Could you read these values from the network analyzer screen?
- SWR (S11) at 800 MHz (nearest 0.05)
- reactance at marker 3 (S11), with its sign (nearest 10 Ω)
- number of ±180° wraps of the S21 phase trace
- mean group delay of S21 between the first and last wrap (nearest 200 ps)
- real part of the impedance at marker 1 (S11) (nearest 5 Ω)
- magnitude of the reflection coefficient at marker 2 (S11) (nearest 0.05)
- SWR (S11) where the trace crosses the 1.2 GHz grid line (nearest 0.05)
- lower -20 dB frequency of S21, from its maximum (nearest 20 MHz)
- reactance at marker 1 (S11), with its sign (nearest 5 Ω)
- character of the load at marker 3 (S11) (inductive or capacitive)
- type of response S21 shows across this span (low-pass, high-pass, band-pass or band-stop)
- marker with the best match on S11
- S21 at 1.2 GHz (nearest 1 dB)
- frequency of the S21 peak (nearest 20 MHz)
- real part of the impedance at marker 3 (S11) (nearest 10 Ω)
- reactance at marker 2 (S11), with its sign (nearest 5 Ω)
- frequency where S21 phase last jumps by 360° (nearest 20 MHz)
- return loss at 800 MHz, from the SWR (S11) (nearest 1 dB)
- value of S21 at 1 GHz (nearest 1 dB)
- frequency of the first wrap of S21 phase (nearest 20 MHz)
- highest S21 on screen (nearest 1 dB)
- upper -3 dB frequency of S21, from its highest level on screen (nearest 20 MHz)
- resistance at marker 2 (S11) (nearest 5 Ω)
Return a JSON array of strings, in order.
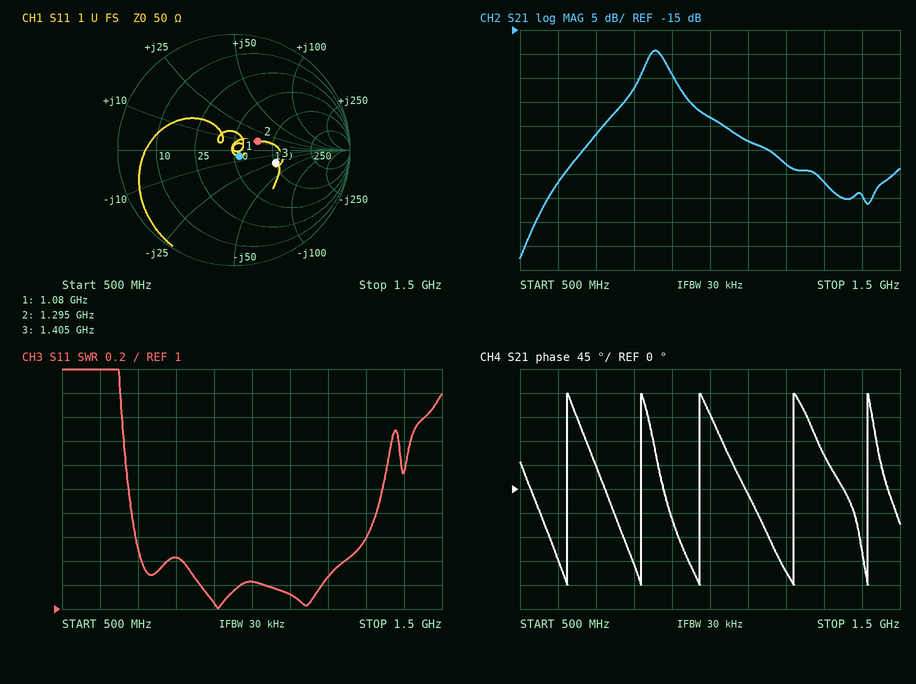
["1.45", "-30 Ω", "5", "5.0 ns", "55 Ω", "0.20", "1.25", "680 MHz", "-5 Ω", "capacitive", "band-pass", "marker 1", "-43 dB", "860 MHz", "100 Ω", "+10 Ω", "1.42 GHz", "15 dB", "-33 dB", "620 MHz", "-19 dB", "880 MHz", "75 Ω"]
